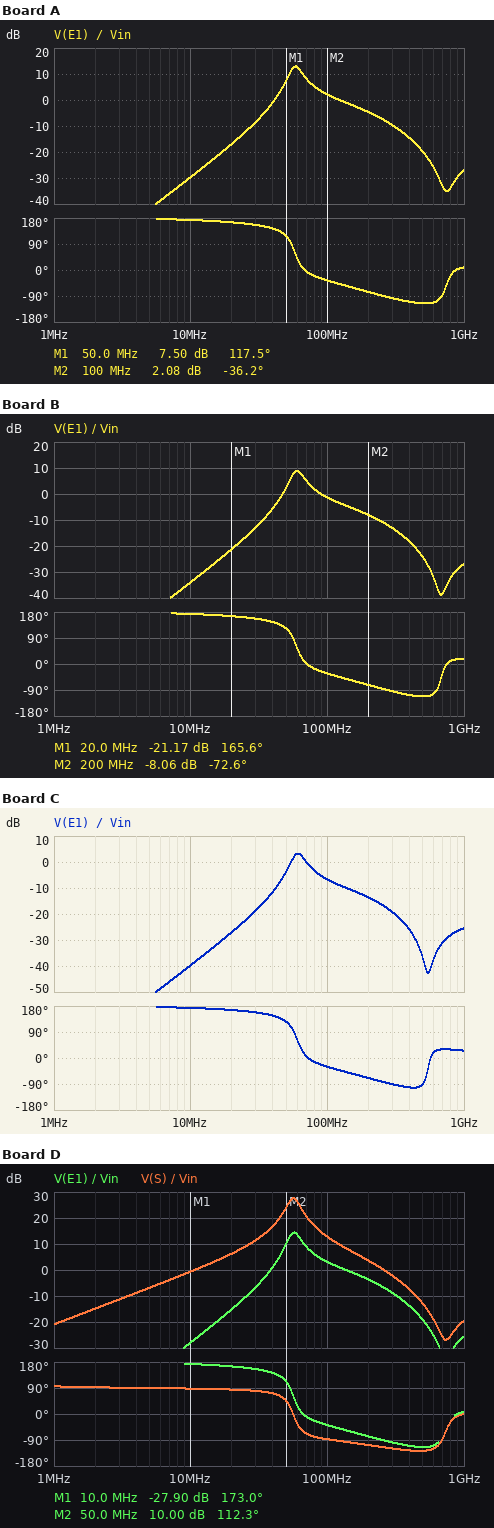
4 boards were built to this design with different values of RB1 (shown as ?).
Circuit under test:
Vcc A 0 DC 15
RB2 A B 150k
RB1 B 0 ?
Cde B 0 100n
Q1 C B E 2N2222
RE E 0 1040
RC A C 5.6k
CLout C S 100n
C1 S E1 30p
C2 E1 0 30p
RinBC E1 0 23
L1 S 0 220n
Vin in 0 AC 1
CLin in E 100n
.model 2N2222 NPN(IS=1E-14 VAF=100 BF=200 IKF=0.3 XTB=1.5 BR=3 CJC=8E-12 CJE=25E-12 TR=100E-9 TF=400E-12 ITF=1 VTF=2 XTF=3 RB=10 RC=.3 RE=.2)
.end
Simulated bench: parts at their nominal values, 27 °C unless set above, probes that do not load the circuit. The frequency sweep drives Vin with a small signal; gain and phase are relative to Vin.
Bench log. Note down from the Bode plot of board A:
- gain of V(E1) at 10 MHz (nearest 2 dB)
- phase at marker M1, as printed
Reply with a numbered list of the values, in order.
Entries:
1. -30 dB
2. 117.5 deg
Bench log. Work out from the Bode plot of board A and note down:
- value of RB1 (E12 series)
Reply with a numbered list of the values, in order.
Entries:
1. 27 kΩ
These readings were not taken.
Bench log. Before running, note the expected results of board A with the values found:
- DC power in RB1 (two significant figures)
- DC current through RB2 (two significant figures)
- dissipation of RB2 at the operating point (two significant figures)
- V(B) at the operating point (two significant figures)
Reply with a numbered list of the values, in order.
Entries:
1. 170 µW
2. 86 µA
3. 1.1 mW
4. 2.1 V
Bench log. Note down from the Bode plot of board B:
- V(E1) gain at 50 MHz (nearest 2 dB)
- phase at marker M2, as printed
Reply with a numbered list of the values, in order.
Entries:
1. 2 dB
2. -72.6 deg
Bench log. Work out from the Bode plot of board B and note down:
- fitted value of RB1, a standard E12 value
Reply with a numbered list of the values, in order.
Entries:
1. 18 kΩ
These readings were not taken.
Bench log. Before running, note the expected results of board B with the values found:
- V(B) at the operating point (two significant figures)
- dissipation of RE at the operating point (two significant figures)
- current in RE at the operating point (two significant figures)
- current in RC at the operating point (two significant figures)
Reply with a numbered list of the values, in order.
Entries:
1. 1.5 V
2. 770 µW
3. 860 µA
4. 860 µA
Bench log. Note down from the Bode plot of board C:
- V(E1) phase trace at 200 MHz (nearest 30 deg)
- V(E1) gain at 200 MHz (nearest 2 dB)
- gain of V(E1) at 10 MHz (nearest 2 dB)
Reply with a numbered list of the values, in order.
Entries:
1. -60 deg
2. -14 dB
3. -40 dB
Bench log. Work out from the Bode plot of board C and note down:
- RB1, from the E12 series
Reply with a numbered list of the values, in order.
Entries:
1. 12 kΩ
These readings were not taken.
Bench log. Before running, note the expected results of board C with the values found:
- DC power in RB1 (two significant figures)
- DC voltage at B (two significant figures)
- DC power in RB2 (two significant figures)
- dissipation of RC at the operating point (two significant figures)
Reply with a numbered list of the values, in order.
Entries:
1. 99 µW
2. 1.1 V
3. 1.3 mW
4. 1.1 mW
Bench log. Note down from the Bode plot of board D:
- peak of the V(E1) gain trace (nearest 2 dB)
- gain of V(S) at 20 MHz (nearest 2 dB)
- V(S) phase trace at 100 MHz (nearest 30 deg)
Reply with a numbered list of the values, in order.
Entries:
1. 14 dB
2. 6 dB
3. -90 deg
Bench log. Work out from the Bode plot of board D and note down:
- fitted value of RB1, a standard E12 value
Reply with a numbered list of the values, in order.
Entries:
1. 33 kΩ
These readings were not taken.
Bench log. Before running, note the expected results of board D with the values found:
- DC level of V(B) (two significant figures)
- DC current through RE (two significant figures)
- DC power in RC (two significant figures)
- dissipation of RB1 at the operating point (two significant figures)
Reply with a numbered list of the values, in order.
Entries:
1. 2.5 V
2. 1.7 mA
3. 17 mW
4. 190 µW
